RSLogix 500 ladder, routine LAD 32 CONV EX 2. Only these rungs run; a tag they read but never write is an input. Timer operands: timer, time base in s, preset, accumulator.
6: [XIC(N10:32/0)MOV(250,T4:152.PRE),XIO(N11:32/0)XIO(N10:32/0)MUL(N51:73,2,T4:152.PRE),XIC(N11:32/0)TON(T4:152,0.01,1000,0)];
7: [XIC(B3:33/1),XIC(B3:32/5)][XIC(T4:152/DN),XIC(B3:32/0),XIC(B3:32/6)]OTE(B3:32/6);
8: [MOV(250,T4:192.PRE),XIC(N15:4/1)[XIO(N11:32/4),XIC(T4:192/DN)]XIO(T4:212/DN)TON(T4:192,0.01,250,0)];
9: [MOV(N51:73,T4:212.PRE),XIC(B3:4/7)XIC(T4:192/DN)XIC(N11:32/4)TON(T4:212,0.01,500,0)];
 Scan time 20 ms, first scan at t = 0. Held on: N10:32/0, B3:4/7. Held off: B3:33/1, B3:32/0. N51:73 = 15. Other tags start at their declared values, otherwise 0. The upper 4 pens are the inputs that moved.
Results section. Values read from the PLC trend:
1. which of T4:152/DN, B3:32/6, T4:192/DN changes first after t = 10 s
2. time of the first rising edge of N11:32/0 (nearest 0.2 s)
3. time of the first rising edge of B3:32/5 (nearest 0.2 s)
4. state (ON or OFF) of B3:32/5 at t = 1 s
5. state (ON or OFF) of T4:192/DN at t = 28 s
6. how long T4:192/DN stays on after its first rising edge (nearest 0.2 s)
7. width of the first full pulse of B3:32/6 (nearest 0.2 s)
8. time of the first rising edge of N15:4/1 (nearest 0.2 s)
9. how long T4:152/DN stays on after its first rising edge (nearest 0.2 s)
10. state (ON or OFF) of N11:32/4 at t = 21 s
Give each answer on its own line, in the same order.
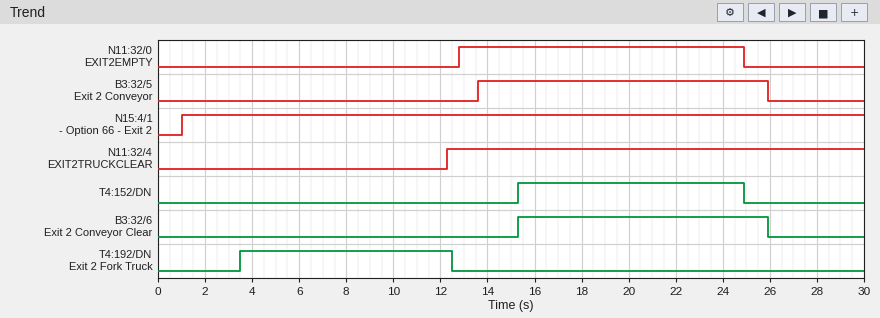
T4:192/DN
12.8 s
13.6 s
OFF
OFF
9.0 s
10.6 s
1.0 s
9.6 s
ON
